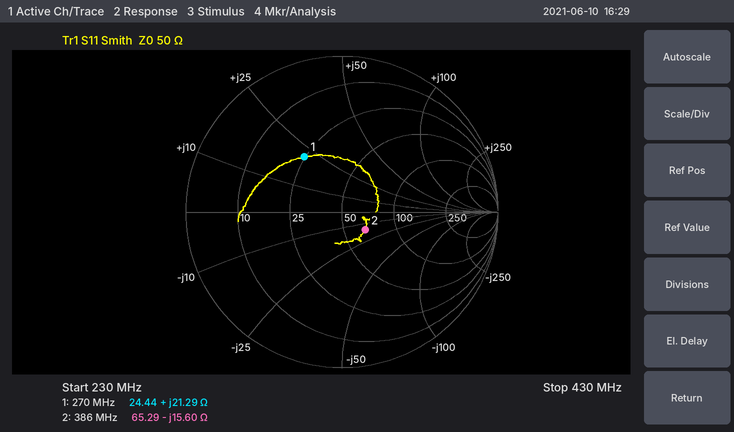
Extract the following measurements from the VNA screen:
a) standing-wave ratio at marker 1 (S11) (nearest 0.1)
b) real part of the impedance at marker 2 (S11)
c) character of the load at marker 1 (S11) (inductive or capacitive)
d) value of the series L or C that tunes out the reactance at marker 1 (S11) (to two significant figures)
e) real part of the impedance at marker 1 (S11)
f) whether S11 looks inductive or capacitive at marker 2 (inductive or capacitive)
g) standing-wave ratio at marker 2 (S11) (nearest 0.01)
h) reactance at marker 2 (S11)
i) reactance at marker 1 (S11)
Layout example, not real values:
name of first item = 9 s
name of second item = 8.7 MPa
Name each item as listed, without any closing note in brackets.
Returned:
standing-wave ratio at marker 1 (S11) = 2.5
real part of the impedance at marker 2 = 65.29 Ω
character of the load at marker 1 (S11) = inductive
value of the series L or C that tunes out the reactance at marker 1 (S11) = 28 pF
real part of the impedance at marker 1 = 24.44 Ω
whether S11 looks inductive or capacitive at marker 2 = capacitive
standing-wave ratio at marker 2 (S11) = 1.46
reactance at marker 2 = -15.60 Ω
reactance at marker 1 = +21.29 Ω
